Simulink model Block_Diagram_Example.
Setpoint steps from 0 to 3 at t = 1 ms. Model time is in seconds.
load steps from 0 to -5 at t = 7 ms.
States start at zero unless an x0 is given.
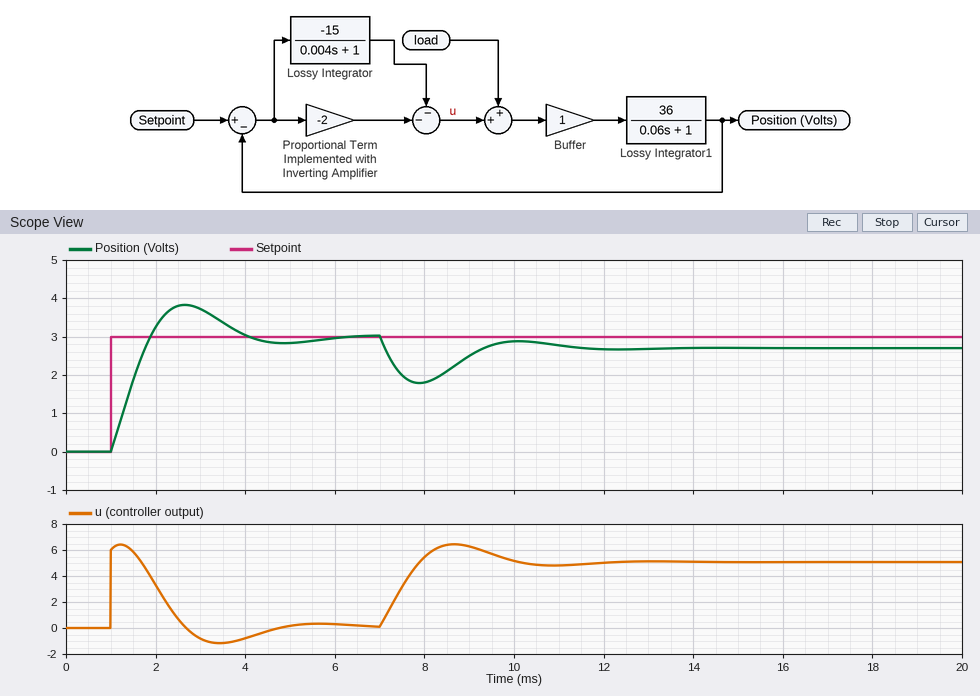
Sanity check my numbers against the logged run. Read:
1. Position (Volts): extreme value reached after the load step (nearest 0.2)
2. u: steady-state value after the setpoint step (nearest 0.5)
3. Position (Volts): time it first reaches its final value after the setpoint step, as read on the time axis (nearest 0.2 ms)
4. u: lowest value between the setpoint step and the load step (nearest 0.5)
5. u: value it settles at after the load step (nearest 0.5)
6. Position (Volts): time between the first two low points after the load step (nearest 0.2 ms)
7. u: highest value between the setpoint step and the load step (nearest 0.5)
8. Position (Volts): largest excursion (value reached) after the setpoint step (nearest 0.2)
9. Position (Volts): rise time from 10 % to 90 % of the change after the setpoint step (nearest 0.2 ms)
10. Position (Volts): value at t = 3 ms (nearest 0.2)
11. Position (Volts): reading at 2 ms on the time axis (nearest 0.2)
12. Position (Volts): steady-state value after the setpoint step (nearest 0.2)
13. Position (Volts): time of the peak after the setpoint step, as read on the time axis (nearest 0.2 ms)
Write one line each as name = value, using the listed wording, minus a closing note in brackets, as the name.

Position (Volts): extreme value reached after the load step = 1.8
u: steady-state value after the setpoint step = 0.0
Position (Volts): time it first reaches its final value after the setpoint step, as read on the time axis = 1.8 ms
u: lowest value between the setpoint step and the load step = -1.0
u: value it settles at after the load step = 5.0
Position (Volts): time between the first two low points after the load step = 4.4 ms
u: highest value between the setpoint step and the load step = 6.5
Position (Volts): largest excursion (value reached) after the setpoint step = 3.8
Position (Volts): rise time from 10 % to 90 % of the change after the setpoint step = 0.6 ms
Position (Volts): value at t = 3 ms = 3.8
Position (Volts): reading at 2 ms on the time axis = 3.2
Position (Volts): steady-state value after the setpoint step = 3.0
Position (Volts): time of the peak after the setpoint step, as read on the time axis = 2.6 ms
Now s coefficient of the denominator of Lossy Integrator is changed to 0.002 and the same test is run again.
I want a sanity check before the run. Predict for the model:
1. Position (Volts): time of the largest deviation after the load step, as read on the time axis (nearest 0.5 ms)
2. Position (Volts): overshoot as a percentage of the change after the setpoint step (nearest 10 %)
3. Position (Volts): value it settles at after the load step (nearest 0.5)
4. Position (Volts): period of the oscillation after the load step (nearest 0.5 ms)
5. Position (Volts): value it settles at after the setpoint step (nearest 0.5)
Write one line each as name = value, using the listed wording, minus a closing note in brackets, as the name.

Position (Volts): time of the largest deviation after the load step, as read on the time axis = 7.5 ms
Position (Volts): overshoot as a percentage of the change after the setpoint step = 30 %
Position (Volts): value it settles at after the load step = 2.5
Position (Volts): period of the oscillation after the load step = 3.0 ms
Position (Volts): value it settles at after the setpoint step = 3.0
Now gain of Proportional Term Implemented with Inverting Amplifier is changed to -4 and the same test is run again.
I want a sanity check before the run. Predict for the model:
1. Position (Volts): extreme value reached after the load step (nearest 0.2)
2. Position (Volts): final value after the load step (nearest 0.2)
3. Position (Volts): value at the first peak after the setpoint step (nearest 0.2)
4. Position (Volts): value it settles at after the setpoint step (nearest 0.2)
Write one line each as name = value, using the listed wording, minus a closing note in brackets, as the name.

Position (Volts): extreme value reached after the load step = 2.2
Position (Volts): final value after the load step = 2.8
Position (Volts): value at the first peak after the setpoint step = 3.4
Position (Volts): value it settles at after the setpoint step = 3.0
